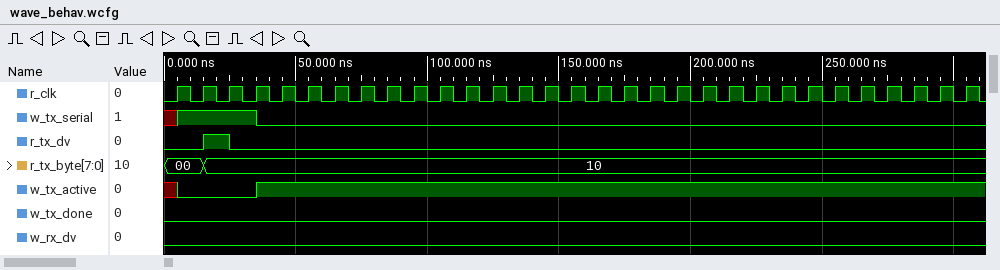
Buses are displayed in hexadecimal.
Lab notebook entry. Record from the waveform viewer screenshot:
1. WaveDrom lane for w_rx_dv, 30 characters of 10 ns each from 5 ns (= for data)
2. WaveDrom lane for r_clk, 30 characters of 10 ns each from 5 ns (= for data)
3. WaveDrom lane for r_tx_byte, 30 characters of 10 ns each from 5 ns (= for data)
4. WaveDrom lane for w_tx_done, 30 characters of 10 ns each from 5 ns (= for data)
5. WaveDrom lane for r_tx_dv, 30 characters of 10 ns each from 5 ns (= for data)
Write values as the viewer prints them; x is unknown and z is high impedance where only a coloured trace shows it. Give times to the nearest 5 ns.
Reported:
{name: 'w_rx_dv', wave: '0.............................'}
{name: 'r_clk', wave: 'p.............................'}
{name: 'r_tx_byte', wave: '==............................', data: '00 10'}
{name: 'w_tx_done', wave: '0.............................'}
{name: 'r_tx_dv', wave: '010...........................'}
